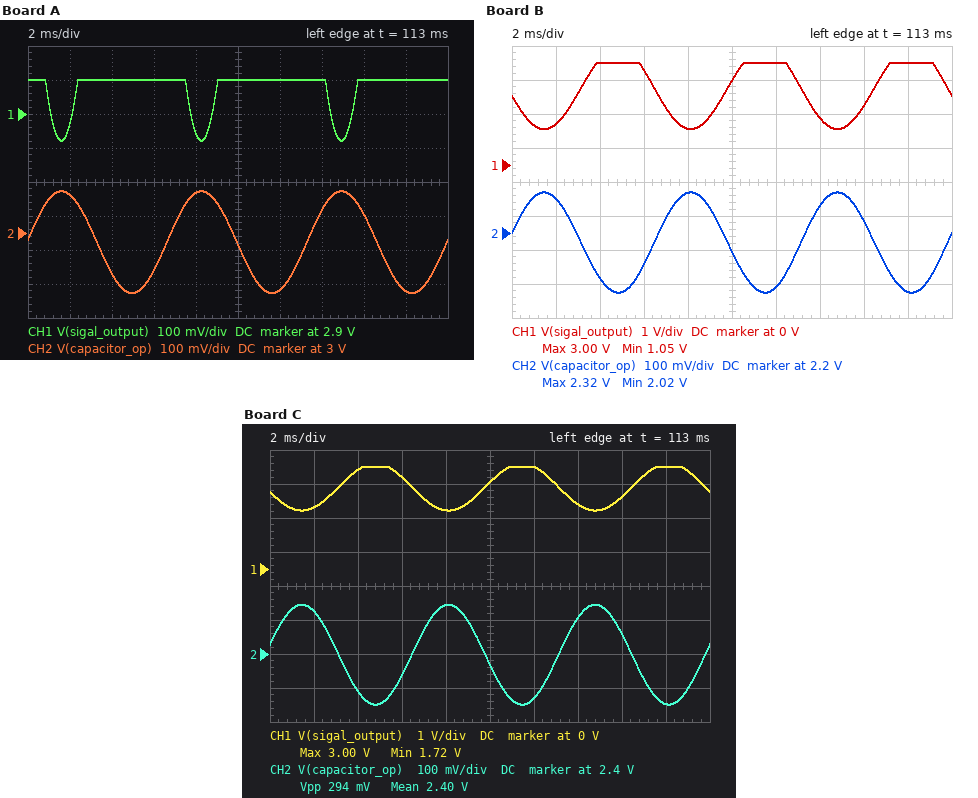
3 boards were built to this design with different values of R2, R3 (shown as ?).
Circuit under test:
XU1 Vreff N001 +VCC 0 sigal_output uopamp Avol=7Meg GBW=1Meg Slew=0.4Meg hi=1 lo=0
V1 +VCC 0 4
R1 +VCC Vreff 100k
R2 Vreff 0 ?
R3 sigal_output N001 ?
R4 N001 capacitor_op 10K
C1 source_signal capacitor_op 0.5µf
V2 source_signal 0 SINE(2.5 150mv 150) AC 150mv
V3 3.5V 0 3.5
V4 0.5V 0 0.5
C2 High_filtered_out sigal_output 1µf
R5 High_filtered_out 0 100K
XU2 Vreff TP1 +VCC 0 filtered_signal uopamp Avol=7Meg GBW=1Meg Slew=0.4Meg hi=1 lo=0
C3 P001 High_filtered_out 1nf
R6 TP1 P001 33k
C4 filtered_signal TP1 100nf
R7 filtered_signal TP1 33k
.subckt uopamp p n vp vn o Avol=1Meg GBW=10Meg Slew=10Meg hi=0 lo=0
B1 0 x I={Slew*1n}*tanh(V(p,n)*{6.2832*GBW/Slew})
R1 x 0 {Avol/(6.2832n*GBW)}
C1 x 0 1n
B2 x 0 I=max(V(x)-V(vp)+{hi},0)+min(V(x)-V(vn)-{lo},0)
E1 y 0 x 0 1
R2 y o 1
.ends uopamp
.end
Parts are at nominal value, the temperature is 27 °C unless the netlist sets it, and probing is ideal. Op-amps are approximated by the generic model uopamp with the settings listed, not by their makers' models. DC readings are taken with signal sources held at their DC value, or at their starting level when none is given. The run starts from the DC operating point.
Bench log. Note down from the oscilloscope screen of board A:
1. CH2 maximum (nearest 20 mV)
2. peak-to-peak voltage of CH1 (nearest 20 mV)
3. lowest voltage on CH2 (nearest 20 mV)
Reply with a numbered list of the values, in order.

1. 3.12 V
2. 180 mV
3. 2.82 V
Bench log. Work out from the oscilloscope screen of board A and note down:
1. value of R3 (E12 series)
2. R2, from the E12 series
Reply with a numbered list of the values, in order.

1. 47 kΩ
2. 330 kΩ
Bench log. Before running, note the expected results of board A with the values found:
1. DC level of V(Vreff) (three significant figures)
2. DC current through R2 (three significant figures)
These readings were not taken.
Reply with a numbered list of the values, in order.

1. 3.07 V
2. 9.30 µA
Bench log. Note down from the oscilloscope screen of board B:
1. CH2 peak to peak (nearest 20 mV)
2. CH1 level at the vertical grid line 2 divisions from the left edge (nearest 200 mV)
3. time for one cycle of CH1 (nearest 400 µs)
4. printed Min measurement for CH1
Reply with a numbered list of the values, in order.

1. 300 mV
2. 3.0 V
3. 6.8 ms
4. 1.05 V
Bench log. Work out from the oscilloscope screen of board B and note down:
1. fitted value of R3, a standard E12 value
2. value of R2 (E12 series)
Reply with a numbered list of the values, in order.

1. 82 kΩ
2. 120 kΩ
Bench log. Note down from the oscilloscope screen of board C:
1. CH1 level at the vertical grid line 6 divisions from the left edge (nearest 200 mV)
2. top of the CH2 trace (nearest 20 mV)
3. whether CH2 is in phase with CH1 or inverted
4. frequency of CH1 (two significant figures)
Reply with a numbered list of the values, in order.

1. 3.0 V
2. 2.54 V
3. inverted
4. 150 Hz
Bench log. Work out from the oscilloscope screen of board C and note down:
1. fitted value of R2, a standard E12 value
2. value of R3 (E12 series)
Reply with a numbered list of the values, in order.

1. 150 kΩ
2. 47 kΩ
